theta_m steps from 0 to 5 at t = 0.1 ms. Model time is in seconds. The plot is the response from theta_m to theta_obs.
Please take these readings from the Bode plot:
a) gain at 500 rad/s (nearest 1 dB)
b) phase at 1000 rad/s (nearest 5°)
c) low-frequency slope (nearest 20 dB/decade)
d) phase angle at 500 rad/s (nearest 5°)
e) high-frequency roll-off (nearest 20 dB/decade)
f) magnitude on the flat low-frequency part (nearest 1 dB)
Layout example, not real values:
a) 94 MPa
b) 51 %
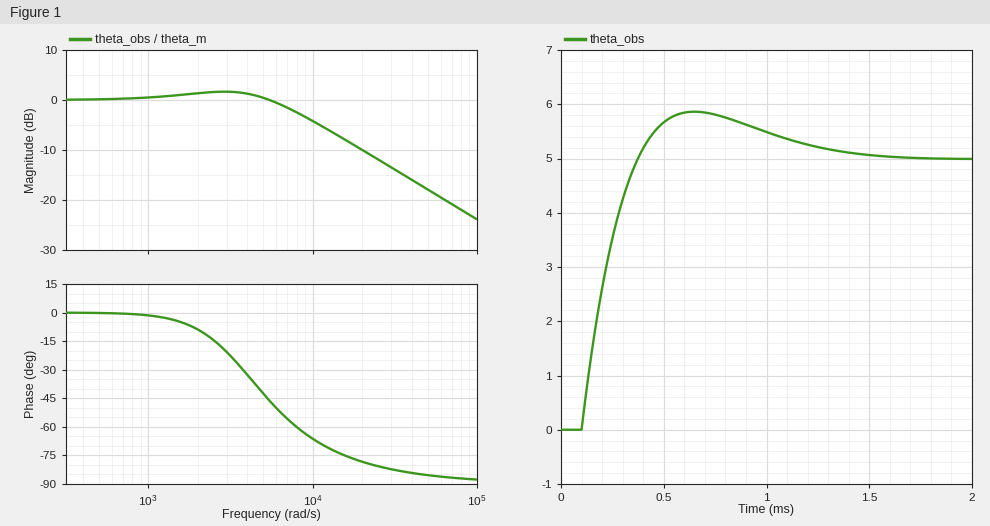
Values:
a) 0 dB
b) 0°
c) 0 dB/decade
d) 0°
e) -20 dB/decade
f) 0 dB
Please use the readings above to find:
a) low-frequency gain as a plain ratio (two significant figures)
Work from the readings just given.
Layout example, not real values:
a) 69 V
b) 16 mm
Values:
a) 1.0
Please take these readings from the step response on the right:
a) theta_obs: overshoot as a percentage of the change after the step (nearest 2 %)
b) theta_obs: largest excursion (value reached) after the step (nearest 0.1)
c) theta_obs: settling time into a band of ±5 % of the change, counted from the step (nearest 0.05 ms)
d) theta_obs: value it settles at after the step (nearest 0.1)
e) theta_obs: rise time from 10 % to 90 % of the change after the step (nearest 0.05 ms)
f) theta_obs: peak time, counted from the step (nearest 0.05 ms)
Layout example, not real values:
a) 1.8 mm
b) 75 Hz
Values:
a) 18 %
b) 5.9
c) 1.10 ms
d) 5.0
e) 0.20 ms
f) 0.55 ms
